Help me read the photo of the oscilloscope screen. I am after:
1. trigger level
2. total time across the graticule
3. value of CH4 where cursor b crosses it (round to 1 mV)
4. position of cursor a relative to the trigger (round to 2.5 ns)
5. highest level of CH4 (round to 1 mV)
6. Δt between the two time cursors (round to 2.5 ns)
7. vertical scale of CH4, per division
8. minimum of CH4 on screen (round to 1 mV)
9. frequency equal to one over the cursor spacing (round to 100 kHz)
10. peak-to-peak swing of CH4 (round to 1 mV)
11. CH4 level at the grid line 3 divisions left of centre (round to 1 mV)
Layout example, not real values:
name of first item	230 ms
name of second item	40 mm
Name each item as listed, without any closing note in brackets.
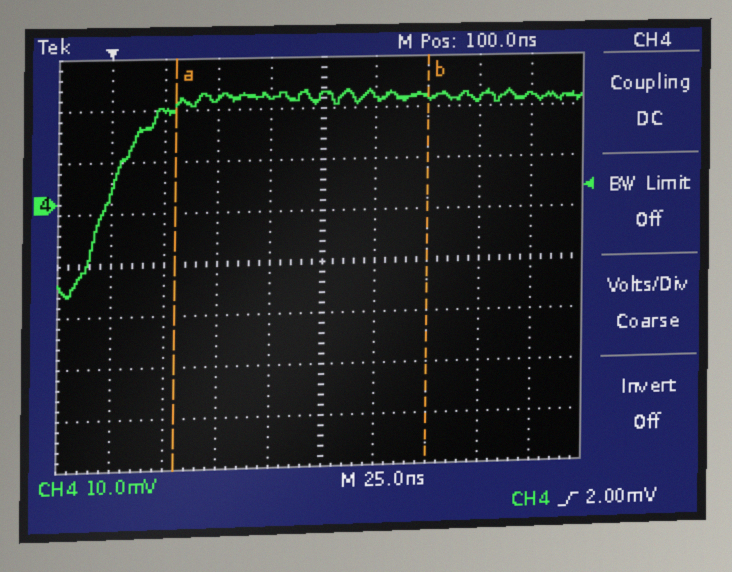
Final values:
trigger level	2.00 mV
total time across the graticule	250 ns
value of CH4 where cursor b crosses it	20 mV
position of cursor a relative to the trigger	+30.0 ns
highest level of CH4	22 mV
Δt between the two time cursors	120.0 ns
vertical scale of CH4, per division	10 mV
minimum of CH4 on screen	-18 mV
frequency equal to one over the cursor spacing	8.3 MHz
peak-to-peak swing of CH4	40 mV
CH4 level at the grid line 3 divisions left of centre	18 mV
